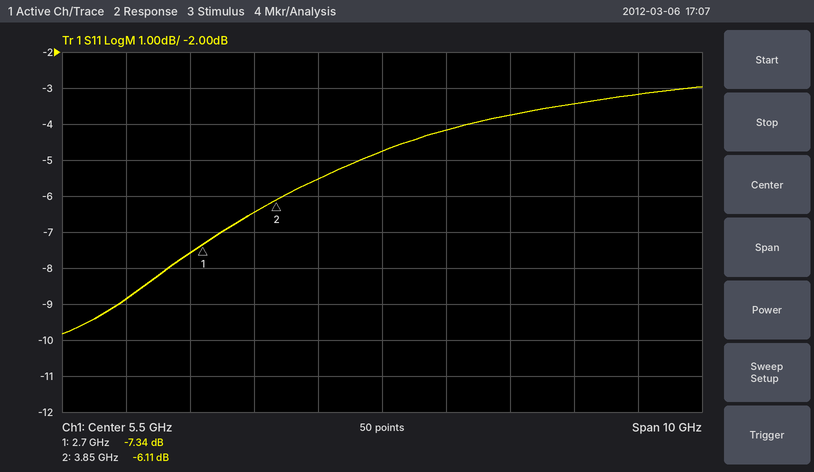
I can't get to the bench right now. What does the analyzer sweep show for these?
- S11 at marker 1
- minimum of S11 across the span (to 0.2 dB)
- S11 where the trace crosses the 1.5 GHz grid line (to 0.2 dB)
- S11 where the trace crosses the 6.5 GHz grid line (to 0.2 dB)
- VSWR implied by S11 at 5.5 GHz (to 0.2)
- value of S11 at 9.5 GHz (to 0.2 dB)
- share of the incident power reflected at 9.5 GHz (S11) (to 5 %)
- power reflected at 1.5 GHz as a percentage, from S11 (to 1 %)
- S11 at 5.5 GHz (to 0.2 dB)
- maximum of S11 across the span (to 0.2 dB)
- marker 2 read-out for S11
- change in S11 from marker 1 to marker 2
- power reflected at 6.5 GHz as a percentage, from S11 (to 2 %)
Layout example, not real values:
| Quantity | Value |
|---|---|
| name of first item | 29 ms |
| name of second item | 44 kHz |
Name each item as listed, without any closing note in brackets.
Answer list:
| Quantity | Value |
|---|---|
| S11 at marker 1 | -7.34 dB |
| minimum of S11 across the span | -9.8 dB |
| S11 where the trace crosses the 1.5 GHz grid line | -8.8 dB |
| S11 where the trace crosses the 6.5 GHz grid line | -4.2 dB |
| VSWR implied by S11 at 5.5 GHz | 3.8 |
| value of S11 at 9.5 GHz | -3.2 dB |
| share of the incident power reflected at 9.5 GHz (S11) | 50 % |
| power reflected at 1.5 GHz as a percentage, from S11 | 13 % |
| S11 at 5.5 GHz | -4.8 dB |
| maximum of S11 across the span | -3.0 dB |
| marker 2 read-out for S11 | -6.11 dB |
| change in S11 from marker 1 to marker 2 | 1.23 dB |
| power reflected at 6.5 GHz as a percentage, from S11 | 38 % |
